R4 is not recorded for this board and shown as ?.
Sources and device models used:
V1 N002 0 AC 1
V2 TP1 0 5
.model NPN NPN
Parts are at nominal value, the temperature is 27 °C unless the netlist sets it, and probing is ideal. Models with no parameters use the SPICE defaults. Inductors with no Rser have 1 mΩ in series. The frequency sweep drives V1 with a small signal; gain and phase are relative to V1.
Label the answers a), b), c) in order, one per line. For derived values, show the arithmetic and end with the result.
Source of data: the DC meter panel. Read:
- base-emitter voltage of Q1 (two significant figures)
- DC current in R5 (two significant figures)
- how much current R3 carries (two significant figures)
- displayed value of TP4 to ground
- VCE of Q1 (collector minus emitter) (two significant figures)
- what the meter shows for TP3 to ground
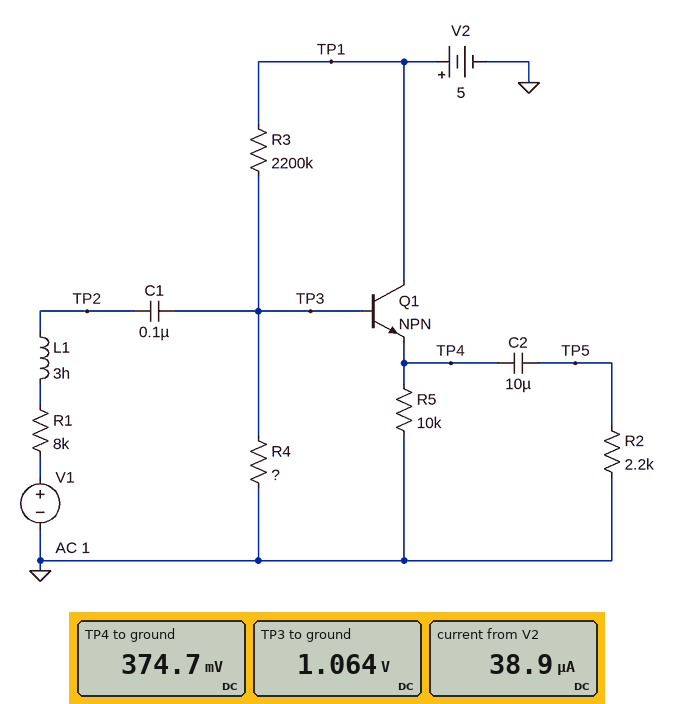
a) 1.064 V - 374.7 mV = 690 mV
b) (374.7 mV) / 10 kΩ = 37 µA
c) (5 V - 1.064 V) / 2.2 MΩ = 1.8 µA
d) 374.7 mV
e) 5 V - 374.7 mV = 4.6 V
f) 1.064 V
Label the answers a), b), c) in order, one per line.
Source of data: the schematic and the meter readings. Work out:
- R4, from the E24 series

a) 750 kΩ
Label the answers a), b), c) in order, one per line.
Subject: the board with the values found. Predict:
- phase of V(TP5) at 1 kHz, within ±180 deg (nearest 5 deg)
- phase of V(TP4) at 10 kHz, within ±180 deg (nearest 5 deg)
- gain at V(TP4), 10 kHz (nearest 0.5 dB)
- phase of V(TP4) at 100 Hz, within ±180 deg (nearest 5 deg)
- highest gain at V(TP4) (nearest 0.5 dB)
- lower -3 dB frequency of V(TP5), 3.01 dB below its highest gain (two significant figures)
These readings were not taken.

a) -5 deg
b) -45 deg
c) -6.5 dB
d) 5 deg
e) -3.0 dB
f) 13 Hz
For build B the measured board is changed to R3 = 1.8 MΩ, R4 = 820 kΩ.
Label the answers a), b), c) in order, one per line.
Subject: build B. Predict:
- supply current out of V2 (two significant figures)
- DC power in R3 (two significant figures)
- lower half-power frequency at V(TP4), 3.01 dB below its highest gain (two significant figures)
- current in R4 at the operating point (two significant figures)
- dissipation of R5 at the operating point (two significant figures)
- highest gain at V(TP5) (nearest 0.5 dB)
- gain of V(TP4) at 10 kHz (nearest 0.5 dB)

a) 57 µA
b) 7.8 µW
c) 9.1 Hz
d) 1.5 µA
e) 31 µW
f) -2.5 dB
g) -6.0 dB
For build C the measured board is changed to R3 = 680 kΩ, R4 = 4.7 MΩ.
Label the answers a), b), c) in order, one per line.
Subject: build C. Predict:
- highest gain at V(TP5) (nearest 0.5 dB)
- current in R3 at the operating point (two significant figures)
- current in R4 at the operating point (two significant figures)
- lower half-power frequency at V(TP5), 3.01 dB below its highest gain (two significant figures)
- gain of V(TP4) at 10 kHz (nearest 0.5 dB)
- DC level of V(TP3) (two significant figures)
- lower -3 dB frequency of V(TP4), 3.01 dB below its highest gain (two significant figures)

a) -1.0 dB
b) 2.9 µA
c) 640 nA
d) 15 Hz
e) -5.0 dB
f) 3.0 V
g) 12 Hz
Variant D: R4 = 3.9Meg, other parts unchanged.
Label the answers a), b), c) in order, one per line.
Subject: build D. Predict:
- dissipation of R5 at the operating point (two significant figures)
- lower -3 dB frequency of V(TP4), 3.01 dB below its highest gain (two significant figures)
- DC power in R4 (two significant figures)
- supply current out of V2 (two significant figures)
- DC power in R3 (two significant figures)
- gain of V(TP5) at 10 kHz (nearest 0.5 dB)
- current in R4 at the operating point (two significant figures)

a) 110 µW
b) 9.1 Hz
c) 790 nW
d) 100 µA
e) 4.8 µW
f) -4.5 dB
g) 450 nA
